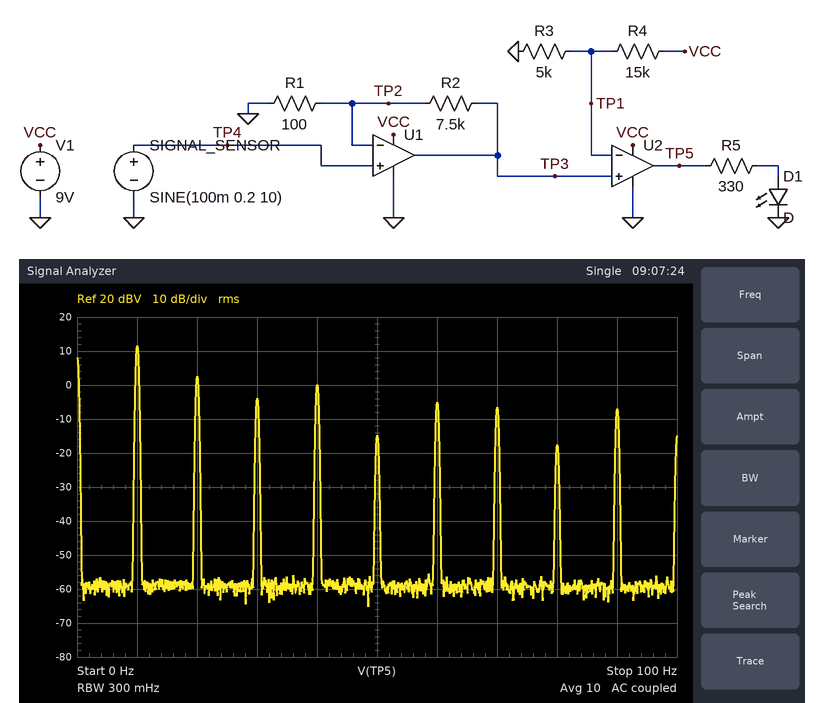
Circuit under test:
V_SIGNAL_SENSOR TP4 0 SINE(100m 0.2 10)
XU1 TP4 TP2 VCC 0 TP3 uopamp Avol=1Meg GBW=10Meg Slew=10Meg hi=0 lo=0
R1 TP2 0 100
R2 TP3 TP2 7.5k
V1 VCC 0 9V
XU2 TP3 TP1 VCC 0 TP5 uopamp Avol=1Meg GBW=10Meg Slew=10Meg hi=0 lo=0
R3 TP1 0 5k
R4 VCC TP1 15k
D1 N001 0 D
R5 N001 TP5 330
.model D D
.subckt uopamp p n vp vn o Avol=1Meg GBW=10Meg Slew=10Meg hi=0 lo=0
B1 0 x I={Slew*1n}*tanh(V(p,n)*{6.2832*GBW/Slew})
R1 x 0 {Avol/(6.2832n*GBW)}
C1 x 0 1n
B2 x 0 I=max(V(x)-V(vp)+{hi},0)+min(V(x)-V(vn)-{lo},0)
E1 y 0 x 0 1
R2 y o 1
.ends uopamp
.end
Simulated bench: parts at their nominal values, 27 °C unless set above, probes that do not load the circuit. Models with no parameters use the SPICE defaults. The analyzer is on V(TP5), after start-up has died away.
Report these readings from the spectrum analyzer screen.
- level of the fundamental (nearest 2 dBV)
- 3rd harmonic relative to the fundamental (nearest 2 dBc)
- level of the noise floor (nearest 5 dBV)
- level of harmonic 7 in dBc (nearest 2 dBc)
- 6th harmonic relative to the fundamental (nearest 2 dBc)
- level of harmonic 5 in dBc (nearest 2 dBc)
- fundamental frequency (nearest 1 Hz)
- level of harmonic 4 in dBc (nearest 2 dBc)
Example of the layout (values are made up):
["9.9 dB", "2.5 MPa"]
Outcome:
["12 dBV", "-16 dBc", "-60 dBV", "-18 dBc", "-16 dBc", "-26 dBc", "10 Hz", "-12 dBc"]
